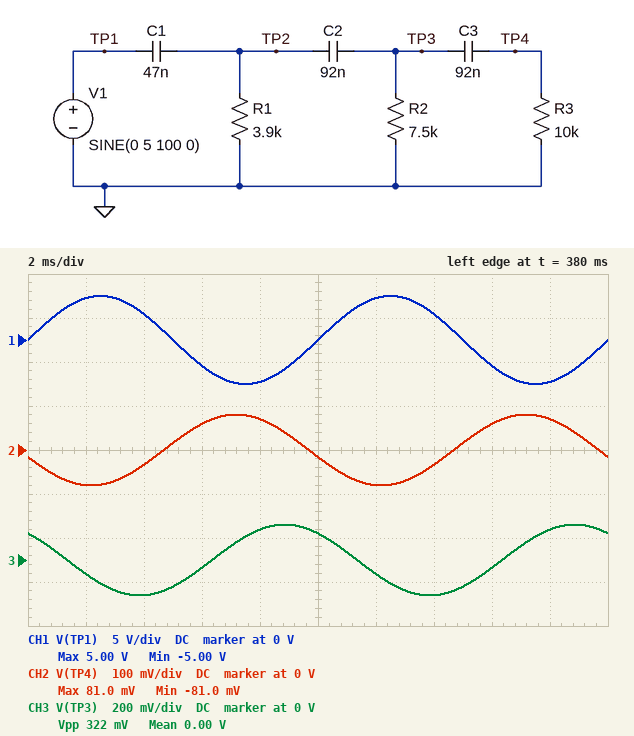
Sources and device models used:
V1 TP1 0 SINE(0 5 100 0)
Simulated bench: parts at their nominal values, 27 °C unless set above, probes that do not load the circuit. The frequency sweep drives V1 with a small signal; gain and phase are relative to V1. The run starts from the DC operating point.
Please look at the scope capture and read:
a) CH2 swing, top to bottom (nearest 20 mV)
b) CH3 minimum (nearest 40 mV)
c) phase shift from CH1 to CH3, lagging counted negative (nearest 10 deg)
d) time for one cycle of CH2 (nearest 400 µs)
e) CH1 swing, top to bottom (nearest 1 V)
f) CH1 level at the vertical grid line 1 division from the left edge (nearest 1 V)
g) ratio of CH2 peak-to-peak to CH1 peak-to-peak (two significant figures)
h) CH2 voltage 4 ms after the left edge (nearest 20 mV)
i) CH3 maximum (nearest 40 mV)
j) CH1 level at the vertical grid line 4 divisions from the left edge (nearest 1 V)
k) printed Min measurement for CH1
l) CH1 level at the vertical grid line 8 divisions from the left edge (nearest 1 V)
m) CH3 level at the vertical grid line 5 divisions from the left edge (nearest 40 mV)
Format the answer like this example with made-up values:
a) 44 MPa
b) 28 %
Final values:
a) 160 mV
b) -160 mV
c) 130 deg
d) 10.0 ms
e) 10 V
f) 5 V
g) 0.016
h) -40 mV
i) 160 mV
j) -5 V
k) -5.00 V
l) -3 V
m) 120 mV
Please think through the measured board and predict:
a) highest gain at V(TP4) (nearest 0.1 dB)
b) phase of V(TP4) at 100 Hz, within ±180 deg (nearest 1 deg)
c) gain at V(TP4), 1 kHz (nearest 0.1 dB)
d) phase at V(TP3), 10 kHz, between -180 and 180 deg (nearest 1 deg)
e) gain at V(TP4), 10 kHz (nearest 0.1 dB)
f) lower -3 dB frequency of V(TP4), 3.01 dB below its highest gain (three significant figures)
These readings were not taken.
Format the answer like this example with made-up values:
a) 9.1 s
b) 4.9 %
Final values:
a) 0 dB
b) -169 deg
c) -7.0 dB
d) 12 deg
e) -0.2 dB
f) 1.95 kHz
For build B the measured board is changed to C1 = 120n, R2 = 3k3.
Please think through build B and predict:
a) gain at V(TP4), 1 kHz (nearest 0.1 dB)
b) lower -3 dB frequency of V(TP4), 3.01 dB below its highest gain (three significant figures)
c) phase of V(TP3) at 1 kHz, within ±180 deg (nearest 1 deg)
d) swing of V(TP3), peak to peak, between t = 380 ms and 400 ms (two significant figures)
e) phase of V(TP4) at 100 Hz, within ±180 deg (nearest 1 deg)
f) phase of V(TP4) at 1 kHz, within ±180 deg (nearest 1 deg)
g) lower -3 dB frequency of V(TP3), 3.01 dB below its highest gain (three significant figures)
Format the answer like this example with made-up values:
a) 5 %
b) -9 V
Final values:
a) -5.1 dB
b) 1.48 kHz
c) 63 deg
d) 430 mV
e) -163 deg
f) 72 deg
g) 1.46 kHz
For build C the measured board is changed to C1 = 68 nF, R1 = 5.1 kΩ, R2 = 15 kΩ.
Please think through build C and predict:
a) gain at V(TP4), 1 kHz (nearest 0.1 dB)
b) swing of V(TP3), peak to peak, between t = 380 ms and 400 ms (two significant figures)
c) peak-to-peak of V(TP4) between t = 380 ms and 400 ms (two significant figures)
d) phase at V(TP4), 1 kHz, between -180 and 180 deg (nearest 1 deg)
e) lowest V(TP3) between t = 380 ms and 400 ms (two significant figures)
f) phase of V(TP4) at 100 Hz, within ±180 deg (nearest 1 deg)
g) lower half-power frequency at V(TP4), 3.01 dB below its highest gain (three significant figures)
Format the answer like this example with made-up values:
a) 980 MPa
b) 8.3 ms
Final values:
a) -3.5 dB
b) 790 mV
c) 400 mV
d) 60 deg
e) -400 mV
f) 171 deg
g) 1.11 kHz
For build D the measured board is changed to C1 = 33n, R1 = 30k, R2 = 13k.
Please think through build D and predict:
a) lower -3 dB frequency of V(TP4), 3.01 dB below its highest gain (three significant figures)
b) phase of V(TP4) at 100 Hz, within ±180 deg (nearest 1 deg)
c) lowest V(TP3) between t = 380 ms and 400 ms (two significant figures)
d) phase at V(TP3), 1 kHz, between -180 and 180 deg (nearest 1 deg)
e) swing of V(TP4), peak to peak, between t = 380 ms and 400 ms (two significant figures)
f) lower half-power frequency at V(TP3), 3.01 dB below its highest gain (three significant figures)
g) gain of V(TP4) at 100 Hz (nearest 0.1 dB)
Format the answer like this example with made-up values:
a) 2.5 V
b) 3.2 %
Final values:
a) 1.38 kHz
b) 144 deg
c) -520 mV
d) 51 deg
e) 520 mV
f) 1.36 kHz
g) -25.6 dB
